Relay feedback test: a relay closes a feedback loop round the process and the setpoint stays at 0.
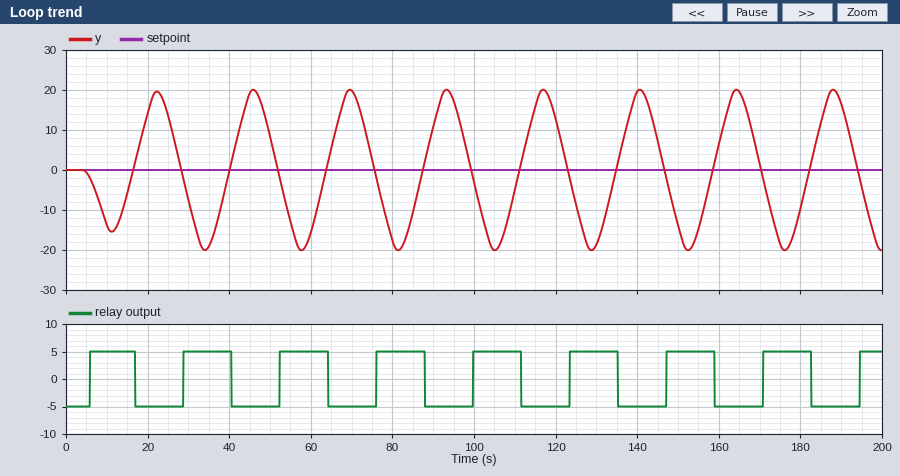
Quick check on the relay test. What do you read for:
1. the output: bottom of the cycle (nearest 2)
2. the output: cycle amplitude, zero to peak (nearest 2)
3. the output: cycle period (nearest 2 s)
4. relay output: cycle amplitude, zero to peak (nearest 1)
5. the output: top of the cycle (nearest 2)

-20
20
24 s
5
20
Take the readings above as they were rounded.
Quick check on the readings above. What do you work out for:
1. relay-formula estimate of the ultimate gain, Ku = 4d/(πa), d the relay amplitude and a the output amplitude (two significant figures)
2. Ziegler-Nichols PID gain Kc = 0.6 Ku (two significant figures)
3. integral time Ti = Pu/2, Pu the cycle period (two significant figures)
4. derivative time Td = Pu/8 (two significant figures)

0.32
0.19
12 s
3.0 s
